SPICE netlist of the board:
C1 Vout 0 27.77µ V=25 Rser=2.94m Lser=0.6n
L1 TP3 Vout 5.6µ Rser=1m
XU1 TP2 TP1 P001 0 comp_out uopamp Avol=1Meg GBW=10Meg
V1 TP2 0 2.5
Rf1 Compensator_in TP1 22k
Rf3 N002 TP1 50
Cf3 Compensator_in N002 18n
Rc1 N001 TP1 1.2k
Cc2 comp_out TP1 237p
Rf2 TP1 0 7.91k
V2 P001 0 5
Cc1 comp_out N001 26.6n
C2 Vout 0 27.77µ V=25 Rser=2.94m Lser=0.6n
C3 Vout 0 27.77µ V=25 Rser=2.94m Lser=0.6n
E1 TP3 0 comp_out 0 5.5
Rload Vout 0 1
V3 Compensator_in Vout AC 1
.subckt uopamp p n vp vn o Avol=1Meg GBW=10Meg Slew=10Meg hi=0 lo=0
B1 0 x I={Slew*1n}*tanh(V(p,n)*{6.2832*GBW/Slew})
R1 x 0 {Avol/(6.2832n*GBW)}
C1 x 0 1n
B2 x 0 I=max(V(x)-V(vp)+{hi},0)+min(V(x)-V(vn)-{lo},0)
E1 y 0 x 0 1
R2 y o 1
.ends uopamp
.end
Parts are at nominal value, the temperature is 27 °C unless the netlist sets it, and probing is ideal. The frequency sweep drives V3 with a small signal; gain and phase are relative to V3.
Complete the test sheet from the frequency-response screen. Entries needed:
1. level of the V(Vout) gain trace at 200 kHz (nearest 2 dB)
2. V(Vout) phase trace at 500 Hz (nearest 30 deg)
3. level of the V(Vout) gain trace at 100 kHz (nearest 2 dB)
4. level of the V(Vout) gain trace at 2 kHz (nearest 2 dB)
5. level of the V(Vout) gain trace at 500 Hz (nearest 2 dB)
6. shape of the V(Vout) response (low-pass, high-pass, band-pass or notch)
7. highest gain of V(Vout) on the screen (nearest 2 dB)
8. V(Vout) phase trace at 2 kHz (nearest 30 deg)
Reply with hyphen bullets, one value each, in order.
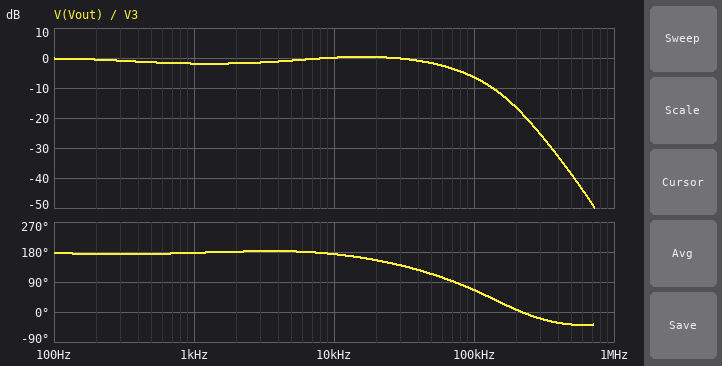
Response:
- -16 dB
- 180 deg
- -6 dB
- -2 dB
- -2 dB
- low-pass
- 0 dB
- 180 deg
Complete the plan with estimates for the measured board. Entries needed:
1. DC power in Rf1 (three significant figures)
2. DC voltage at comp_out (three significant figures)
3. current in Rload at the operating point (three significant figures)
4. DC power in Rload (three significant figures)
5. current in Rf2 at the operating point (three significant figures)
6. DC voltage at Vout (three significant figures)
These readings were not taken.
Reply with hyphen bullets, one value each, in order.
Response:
- 2.20 mW
- 1.72 V
- 9.45 A
- 89.4 W
- 316 µA
- 9.45 V
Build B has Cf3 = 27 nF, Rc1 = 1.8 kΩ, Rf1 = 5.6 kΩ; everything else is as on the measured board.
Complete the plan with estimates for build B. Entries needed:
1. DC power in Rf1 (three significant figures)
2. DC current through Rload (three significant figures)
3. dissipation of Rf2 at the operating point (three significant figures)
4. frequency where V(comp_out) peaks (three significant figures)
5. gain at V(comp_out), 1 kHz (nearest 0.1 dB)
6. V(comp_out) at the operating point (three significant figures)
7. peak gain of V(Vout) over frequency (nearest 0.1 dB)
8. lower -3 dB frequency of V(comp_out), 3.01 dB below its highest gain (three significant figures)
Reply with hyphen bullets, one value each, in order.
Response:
- 559 µW
- 4.27 A
- 790 µW
- 108 kHz
- -15.8 dB
- 777 mV
- 4.9 dB
- 86.0 kHz
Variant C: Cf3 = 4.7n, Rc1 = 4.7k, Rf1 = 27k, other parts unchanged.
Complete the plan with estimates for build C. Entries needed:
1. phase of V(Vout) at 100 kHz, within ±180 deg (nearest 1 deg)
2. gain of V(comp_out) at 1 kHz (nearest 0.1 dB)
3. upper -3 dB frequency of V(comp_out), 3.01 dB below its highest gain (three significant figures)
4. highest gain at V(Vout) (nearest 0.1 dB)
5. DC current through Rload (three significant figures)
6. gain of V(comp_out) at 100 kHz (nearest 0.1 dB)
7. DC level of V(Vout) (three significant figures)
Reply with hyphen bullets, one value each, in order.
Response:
- 62 deg
- -18.4 dB
- 370 kHz
- 0 dB
- 11.0 A
- 23.8 dB
- 11.0 V
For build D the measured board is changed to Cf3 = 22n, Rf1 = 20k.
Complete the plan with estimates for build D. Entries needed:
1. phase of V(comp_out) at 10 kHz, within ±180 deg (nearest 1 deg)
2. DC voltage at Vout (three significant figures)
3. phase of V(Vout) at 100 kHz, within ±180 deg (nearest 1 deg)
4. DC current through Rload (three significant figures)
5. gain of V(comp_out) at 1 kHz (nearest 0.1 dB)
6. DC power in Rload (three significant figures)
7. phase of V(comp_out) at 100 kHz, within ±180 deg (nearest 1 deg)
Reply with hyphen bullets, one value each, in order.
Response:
- -29 deg
- 8.82 V
- 62 deg
- 8.82 A
- -16.5 dB
- 77.8 W
- -122 deg
